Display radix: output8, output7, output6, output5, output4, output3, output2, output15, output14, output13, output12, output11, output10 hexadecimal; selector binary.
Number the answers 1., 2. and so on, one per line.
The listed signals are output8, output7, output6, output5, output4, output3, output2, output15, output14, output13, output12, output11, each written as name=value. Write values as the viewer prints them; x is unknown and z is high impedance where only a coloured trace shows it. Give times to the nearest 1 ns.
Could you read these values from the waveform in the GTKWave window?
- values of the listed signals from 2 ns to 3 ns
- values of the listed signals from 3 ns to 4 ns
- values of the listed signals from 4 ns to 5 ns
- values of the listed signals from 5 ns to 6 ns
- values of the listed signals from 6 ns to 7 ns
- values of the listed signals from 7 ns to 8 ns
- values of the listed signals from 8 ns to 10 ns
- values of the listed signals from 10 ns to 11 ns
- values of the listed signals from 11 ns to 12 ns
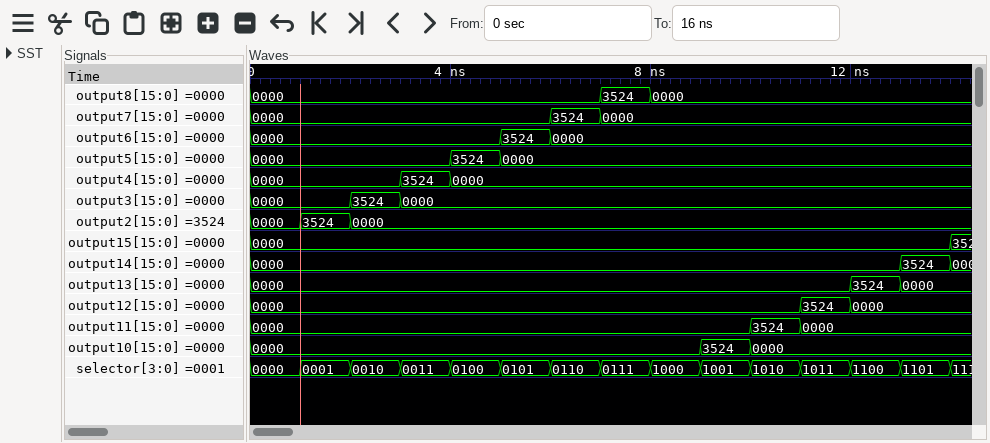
1. output8=0000, output7=0000, output6=0000, output5=0000, output4=0000, output3=3524, output2=0000, output15=0000, output14=0000, output13=0000, output12=0000, output11=0000
2. output8=0000, output7=0000, output6=0000, output5=0000, output4=3524, output3=0000, output2=0000, output15=0000, output14=0000, output13=0000, output12=0000, output11=0000
3. output8=0000, output7=0000, output6=0000, output5=3524, output4=0000, output3=0000, output2=0000, output15=0000, output14=0000, output13=0000, output12=0000, output11=0000
4. output8=0000, output7=0000, output6=3524, output5=0000, output4=0000, output3=0000, output2=0000, output15=0000, output14=0000, output13=0000, output12=0000, output11=0000
5. output8=0000, output7=3524, output6=0000, output5=0000, output4=0000, output3=0000, output2=0000, output15=0000, output14=0000, output13=0000, output12=0000, output11=0000
6. output8=3524, output7=0000, output6=0000, output5=0000, output4=0000, output3=0000, output2=0000, output15=0000, output14=0000, output13=0000, output12=0000, output11=0000
7. output8=0000, output7=0000, output6=0000, output5=0000, output4=0000, output3=0000, output2=0000, output15=0000, output14=0000, output13=0000, output12=0000, output11=0000
8. output8=0000, output7=0000, output6=0000, output5=0000, output4=0000, output3=0000, output2=0000, output15=0000, output14=0000, output13=0000, output12=0000, output11=3524
9. output8=0000, output7=0000, output6=0000, output5=0000, output4=0000, output3=0000, output2=0000, output15=0000, output14=0000, output13=0000, output12=3524, output11=0000
